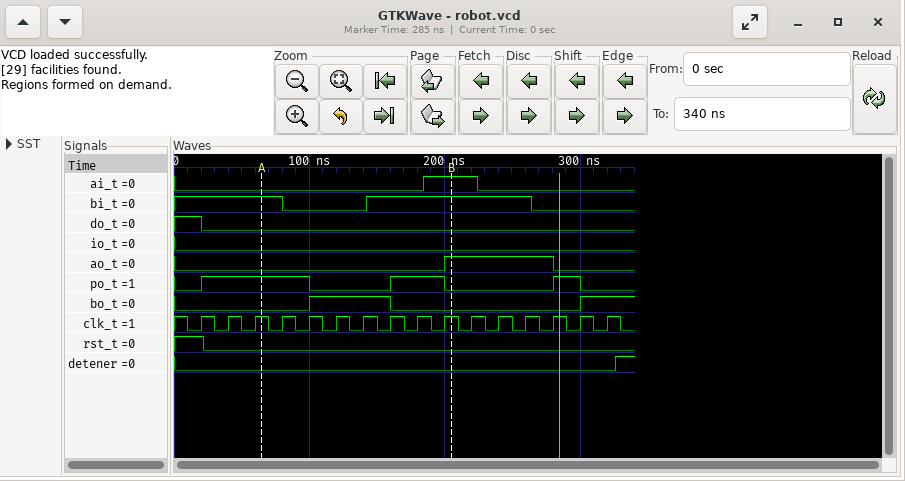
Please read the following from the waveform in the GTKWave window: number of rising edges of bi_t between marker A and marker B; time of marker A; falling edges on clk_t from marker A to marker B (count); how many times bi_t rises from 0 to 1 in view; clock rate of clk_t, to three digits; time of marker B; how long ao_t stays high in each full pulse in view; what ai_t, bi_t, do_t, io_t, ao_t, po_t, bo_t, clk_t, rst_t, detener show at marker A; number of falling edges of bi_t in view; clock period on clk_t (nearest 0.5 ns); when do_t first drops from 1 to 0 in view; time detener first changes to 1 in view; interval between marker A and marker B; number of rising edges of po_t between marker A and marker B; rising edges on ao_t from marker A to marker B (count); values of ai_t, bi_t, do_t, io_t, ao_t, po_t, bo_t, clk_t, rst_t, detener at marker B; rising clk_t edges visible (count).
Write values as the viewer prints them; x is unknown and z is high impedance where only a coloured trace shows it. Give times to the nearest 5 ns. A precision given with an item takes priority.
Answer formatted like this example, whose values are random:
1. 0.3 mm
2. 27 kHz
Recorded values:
1. 1
2. 65 ns
3. 7
4. 1
5. 50.0 MHz
6. 205 ns
7. 80 ns
8. ai_t=0, bi_t=1, do_t=0, io_t=0, ao_t=0, po_t=1, bo_t=0, clk_t=1, rst_t=0, detener=0
9. 2
10. 20 ns
11. 20 ns
12. 325 ns
13. 140 ns
14. 1
15. 1
16. ai_t=1, bi_t=1, do_t=0, io_t=0, ao_t=1, po_t=0, bo_t=0, clk_t=1, rst_t=0, detener=0
17. 16
